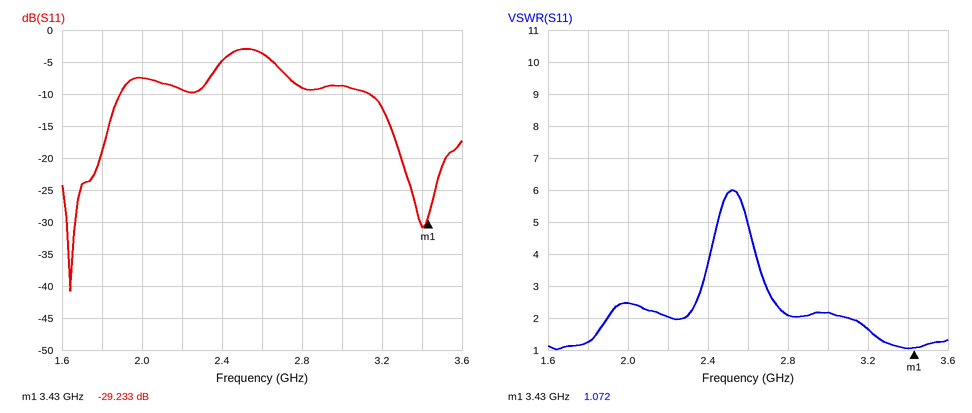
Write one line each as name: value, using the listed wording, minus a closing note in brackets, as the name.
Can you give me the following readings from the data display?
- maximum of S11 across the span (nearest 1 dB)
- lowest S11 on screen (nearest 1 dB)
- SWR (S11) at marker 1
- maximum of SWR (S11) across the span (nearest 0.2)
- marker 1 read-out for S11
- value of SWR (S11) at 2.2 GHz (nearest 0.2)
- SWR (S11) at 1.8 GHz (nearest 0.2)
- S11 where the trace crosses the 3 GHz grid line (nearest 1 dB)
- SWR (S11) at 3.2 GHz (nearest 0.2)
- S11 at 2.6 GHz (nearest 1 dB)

maximum of S11 across the span: -3 dB
lowest S11 on screen: -41 dB
SWR (S11) at marker 1: 1.072
maximum of SWR (S11) across the span: 6.0
marker 1 read-out for S11: -29.233 dB
value of SWR (S11) at 2.2 GHz: 2.0
SWR (S11) at 1.8 GHz: 1.2
S11 where the trace crosses the 3 GHz grid line: -9 dB
SWR (S11) at 3.2 GHz: 1.6
S11 at 2.6 GHz: -4 dB
